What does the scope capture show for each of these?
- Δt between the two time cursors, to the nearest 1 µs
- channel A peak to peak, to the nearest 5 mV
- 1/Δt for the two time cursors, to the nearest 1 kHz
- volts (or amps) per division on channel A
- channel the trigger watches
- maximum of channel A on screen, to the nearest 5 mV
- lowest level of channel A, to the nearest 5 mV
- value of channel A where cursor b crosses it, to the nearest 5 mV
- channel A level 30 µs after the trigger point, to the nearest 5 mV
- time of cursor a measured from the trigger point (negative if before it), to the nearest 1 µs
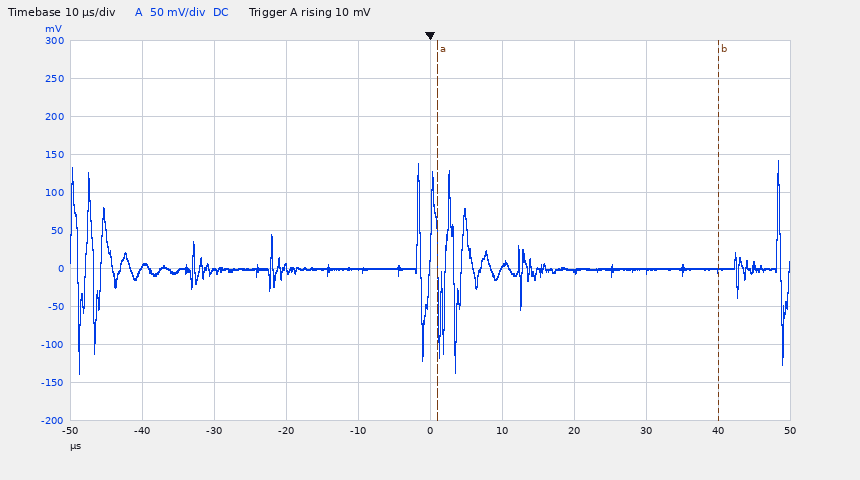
39 µs
280 mV
26 kHz
50 mV
channel A
140 mV
-140 mV
0 mV
-5 mV
+1 µs
